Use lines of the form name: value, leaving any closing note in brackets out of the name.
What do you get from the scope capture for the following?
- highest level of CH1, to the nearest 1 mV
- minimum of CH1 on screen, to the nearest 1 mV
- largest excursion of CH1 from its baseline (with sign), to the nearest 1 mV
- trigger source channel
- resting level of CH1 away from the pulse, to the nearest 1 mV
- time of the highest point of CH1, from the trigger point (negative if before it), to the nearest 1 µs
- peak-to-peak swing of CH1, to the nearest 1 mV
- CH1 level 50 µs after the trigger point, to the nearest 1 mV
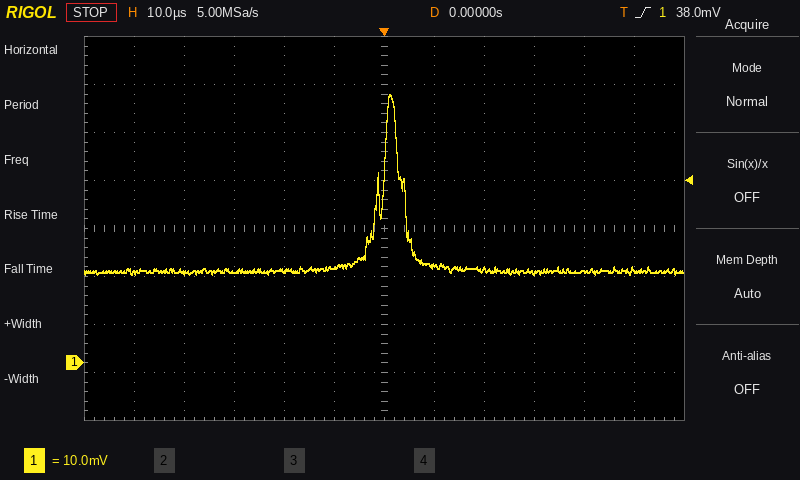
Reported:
highest level of CH1, to the nearest 1 mV: 56 mV
minimum of CH1 on screen, to the nearest 1 mV: 18 mV
largest excursion of CH1 from its baseline (with sign), to the nearest 1 mV: +37 mV
trigger source channel: CH1
resting level of CH1 away from the pulse, to the nearest 1 mV: 19 mV
time of the highest point of CH1, from the trigger point (negative if before it), to the nearest 1 µs: +1 µs
peak-to-peak swing of CH1, to the nearest 1 mV: 38 mV
CH1 level 50 µs after the trigger point, to the nearest 1 mV: 19 mV
